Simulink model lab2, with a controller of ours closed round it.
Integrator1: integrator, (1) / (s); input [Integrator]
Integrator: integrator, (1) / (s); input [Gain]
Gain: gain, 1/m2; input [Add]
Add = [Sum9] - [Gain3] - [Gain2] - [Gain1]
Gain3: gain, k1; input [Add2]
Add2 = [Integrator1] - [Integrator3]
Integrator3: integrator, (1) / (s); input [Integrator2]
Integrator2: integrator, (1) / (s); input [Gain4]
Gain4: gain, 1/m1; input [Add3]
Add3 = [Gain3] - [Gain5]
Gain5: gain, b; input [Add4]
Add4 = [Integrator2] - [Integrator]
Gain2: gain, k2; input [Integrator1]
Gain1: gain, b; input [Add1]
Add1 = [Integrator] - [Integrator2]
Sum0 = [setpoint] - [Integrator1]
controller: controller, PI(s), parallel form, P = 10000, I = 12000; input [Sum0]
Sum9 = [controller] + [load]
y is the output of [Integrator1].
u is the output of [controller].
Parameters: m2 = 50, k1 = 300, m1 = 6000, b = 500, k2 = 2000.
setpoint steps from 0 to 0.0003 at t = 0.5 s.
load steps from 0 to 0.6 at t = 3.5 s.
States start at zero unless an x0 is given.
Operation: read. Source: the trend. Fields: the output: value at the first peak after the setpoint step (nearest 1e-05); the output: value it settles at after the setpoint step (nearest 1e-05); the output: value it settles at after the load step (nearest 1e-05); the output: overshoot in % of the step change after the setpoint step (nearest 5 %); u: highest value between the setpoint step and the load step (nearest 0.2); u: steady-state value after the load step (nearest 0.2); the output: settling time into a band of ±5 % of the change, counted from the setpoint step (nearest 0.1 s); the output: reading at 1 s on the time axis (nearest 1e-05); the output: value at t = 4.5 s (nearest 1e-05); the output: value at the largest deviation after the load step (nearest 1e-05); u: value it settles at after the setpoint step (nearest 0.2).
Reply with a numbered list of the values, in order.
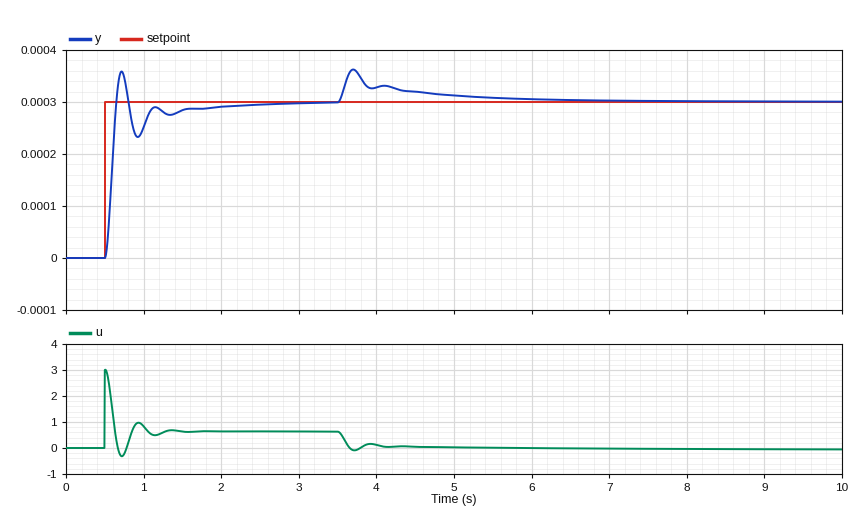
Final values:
1. 0.00036
2. 0.00030
3. 0.00030
4. 20 %
5. 3.0
6. 0.0
7. 1.0 s
8. 0.00025
9. 0.00032
10. 0.00036
11. 0.6
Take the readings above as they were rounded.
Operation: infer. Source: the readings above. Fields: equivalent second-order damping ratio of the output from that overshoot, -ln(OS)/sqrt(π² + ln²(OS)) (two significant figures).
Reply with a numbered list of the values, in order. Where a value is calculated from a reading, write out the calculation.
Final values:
1. ln(0.2) = -1.609; 1.609 / sqrt(9.870 + 2.590) = 0.46
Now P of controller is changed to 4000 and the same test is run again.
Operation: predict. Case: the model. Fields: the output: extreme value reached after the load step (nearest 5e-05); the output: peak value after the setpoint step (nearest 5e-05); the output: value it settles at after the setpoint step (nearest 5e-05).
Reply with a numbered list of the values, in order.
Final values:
1. 0.00040
2. 0.00030
3. 0.00030
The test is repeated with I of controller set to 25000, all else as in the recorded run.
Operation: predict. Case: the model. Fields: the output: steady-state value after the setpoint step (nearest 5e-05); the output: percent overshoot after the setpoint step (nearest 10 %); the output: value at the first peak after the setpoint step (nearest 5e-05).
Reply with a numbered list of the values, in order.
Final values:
1. 0.00030
2. 30 %
3. 0.00040
